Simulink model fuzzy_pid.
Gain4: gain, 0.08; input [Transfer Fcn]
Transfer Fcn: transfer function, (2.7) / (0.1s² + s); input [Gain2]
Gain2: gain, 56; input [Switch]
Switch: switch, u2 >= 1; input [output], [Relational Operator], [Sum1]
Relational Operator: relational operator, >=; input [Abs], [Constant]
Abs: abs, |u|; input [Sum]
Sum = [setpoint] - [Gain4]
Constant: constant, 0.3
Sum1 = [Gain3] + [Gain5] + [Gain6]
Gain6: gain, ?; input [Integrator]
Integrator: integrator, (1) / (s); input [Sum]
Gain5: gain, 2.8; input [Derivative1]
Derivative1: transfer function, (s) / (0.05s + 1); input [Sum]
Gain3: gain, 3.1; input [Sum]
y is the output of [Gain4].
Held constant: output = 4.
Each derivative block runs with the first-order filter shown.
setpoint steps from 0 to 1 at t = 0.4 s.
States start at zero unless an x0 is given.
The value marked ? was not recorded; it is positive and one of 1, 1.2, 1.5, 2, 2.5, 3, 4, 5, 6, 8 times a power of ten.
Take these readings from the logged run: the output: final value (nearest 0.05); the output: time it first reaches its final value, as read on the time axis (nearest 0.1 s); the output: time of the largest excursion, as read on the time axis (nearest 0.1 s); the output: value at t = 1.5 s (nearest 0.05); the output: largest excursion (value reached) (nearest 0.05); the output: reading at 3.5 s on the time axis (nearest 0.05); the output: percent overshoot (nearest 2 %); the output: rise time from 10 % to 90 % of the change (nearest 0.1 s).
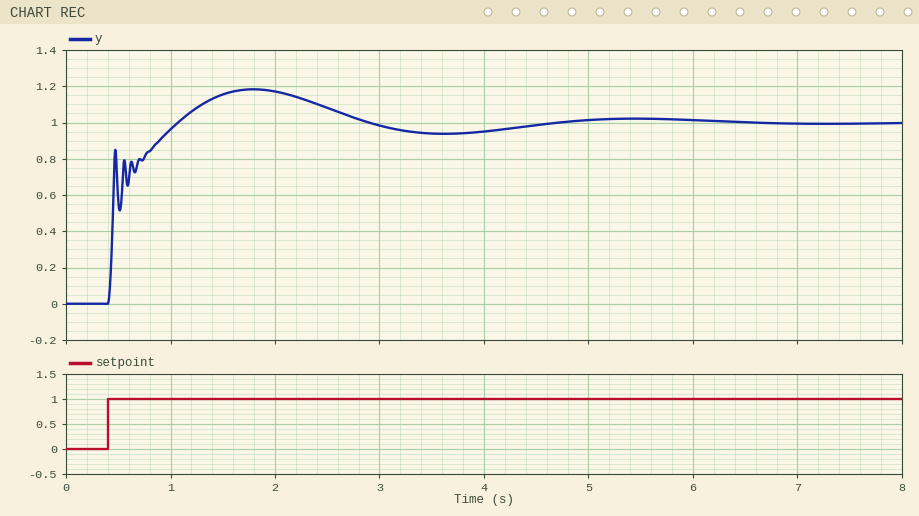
1.00
1.1 s
1.8 s
1.15
1.20
0.95
18 %
0.5 s
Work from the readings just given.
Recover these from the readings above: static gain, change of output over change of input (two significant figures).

1.0
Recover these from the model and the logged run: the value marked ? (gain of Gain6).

10
